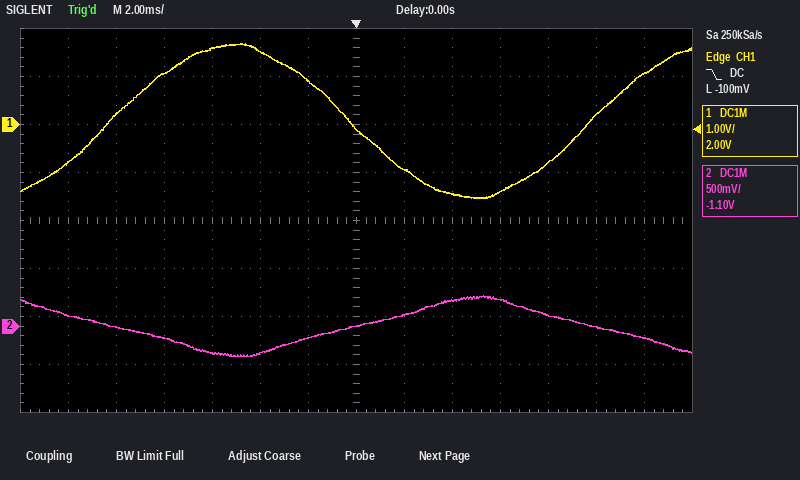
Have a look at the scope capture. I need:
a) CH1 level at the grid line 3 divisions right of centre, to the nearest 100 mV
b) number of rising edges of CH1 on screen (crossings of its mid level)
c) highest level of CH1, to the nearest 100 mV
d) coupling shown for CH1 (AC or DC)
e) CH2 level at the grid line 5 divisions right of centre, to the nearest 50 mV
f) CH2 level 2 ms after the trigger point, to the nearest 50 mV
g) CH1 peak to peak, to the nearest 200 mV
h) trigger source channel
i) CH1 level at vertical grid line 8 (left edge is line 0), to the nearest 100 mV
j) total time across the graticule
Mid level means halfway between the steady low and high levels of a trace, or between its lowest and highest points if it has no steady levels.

-1.4 V
2
1.7 V
DC
0 mV
100 mV
3.2 V
CH1
-900 mV
28 ms
